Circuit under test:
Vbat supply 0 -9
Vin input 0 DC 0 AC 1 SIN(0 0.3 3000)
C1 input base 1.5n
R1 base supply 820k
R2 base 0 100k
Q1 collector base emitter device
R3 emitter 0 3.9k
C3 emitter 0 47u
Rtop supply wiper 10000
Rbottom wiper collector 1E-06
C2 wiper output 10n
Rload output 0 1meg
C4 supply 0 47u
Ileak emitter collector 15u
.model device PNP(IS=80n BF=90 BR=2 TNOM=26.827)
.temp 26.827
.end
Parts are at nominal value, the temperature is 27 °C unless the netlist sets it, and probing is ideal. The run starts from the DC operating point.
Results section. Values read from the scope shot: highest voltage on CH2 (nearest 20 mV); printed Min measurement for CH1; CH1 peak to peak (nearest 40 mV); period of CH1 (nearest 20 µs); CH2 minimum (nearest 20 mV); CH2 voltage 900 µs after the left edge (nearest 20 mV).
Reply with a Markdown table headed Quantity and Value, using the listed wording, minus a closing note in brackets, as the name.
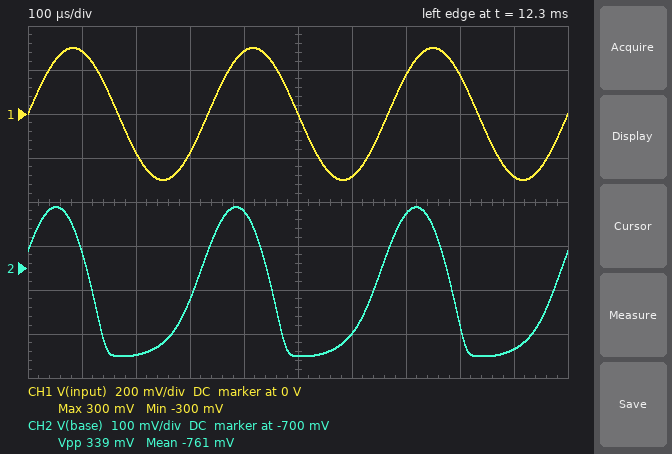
| Quantity | Value |
|---|---|
| highest voltage on CH2 | -560 mV |
| printed Min measurement for CH1 | -300 mV |
| CH1 peak to peak | 600 mV |
| period of CH1 | 340 µs |
| CH2 minimum | -900 mV |
| CH2 voltage 900 µs after the left edge | -880 mV |
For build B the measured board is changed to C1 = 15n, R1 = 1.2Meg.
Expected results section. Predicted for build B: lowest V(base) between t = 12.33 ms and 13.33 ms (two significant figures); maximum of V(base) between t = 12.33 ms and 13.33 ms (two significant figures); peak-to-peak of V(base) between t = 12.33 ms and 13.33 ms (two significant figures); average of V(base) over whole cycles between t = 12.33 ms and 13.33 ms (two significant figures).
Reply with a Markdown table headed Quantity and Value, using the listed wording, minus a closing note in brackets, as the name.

| Quantity | Value |
|---|---|
| lowest V(base) between t = 12.33 ms and 13.33 ms | -680 mV |
| maximum of V(base) between t = 12.33 ms and 13.33 ms | -100 mV |
| peak-to-peak of V(base) between t = 12.33 ms and 13.33 ms | 580 mV |
| average of V(base) over whole cycles between t = 12.33 ms and 13.33 ms | -400 mV |
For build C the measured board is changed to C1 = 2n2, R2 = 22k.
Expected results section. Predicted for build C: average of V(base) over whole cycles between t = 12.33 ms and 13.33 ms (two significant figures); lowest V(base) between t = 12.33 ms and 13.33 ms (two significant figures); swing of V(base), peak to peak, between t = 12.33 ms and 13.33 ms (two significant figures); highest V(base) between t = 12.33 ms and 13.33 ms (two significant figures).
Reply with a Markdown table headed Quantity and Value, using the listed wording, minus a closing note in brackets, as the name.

| Quantity | Value |
|---|---|
| average of V(base) over whole cycles between t = 12.33 ms and 13.33 ms | -210 mV |
| lowest V(base) between t = 12.33 ms and 13.33 ms | -360 mV |
| swing of V(base), peak to peak, between t = 12.33 ms and 13.33 ms | 330 mV |
| highest V(base) between t = 12.33 ms and 13.33 ms | -32 mV |
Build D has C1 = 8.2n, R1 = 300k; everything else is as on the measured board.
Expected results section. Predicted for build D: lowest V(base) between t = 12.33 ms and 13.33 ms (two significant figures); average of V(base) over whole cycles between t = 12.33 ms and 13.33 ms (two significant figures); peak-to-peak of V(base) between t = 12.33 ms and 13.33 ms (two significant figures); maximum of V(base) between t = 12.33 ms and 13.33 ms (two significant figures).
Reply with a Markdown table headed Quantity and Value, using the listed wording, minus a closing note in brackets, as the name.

| Quantity | Value |
|---|---|
| lowest V(base) between t = 12.33 ms and 13.33 ms | -1.9 V |
| average of V(base) over whole cycles between t = 12.33 ms and 13.33 ms | -1.7 V |
| peak-to-peak of V(base) between t = 12.33 ms and 13.33 ms | 460 mV |
| maximum of V(base) between t = 12.33 ms and 13.33 ms | -1.4 V |
